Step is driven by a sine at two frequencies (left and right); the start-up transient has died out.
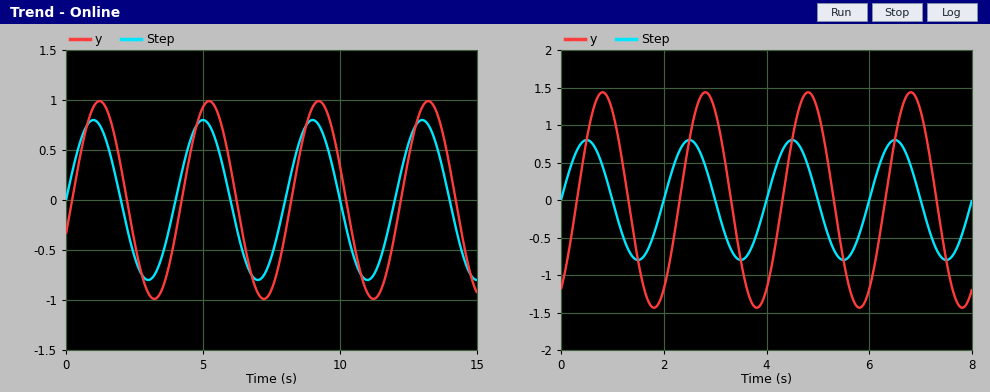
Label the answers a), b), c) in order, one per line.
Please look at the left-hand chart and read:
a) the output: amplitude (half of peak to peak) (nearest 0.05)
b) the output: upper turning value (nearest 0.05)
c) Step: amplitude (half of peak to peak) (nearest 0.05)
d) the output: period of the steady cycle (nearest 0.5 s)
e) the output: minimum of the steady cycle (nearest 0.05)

a) 1.00
b) 1.00
c) 0.80
d) 4.0 s
e) -1.00
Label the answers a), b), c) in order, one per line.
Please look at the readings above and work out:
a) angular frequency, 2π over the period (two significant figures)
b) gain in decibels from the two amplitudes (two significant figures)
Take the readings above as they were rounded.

a) 1.6 rad/s
b) 1.9 dB
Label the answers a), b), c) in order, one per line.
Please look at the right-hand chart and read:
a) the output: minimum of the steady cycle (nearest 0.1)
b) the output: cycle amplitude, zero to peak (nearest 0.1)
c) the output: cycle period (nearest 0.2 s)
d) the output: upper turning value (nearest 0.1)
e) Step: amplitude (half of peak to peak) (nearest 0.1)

a) -1.4
b) 1.4
c) 2.0 s
d) 1.4
e) 0.8
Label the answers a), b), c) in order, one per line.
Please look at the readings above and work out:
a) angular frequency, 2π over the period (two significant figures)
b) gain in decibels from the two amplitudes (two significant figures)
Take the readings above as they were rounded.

a) 3.1 rad/s
b) 4.9 dB
